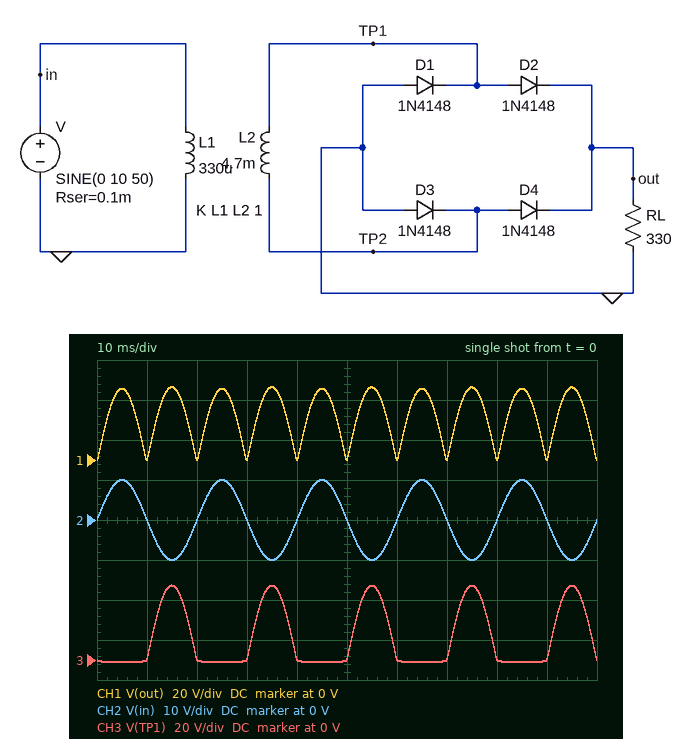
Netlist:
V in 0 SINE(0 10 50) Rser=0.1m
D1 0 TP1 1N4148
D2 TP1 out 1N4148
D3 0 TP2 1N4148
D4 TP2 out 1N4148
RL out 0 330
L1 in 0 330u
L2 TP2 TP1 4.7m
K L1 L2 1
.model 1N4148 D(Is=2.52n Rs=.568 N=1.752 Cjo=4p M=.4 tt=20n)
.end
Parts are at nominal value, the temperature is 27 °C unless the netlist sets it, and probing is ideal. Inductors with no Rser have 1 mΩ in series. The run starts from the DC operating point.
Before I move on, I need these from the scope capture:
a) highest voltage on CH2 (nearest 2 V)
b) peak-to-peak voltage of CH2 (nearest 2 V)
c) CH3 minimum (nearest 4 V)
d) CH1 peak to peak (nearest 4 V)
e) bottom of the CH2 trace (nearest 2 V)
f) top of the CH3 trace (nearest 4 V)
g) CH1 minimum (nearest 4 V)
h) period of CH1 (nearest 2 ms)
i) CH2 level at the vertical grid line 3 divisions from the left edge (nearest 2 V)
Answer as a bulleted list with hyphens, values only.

- 10 V
- 20 V
- 0 V
- 36 V
- -10 V
- 36 V
- 0 V
- 10 ms
- 0 V
